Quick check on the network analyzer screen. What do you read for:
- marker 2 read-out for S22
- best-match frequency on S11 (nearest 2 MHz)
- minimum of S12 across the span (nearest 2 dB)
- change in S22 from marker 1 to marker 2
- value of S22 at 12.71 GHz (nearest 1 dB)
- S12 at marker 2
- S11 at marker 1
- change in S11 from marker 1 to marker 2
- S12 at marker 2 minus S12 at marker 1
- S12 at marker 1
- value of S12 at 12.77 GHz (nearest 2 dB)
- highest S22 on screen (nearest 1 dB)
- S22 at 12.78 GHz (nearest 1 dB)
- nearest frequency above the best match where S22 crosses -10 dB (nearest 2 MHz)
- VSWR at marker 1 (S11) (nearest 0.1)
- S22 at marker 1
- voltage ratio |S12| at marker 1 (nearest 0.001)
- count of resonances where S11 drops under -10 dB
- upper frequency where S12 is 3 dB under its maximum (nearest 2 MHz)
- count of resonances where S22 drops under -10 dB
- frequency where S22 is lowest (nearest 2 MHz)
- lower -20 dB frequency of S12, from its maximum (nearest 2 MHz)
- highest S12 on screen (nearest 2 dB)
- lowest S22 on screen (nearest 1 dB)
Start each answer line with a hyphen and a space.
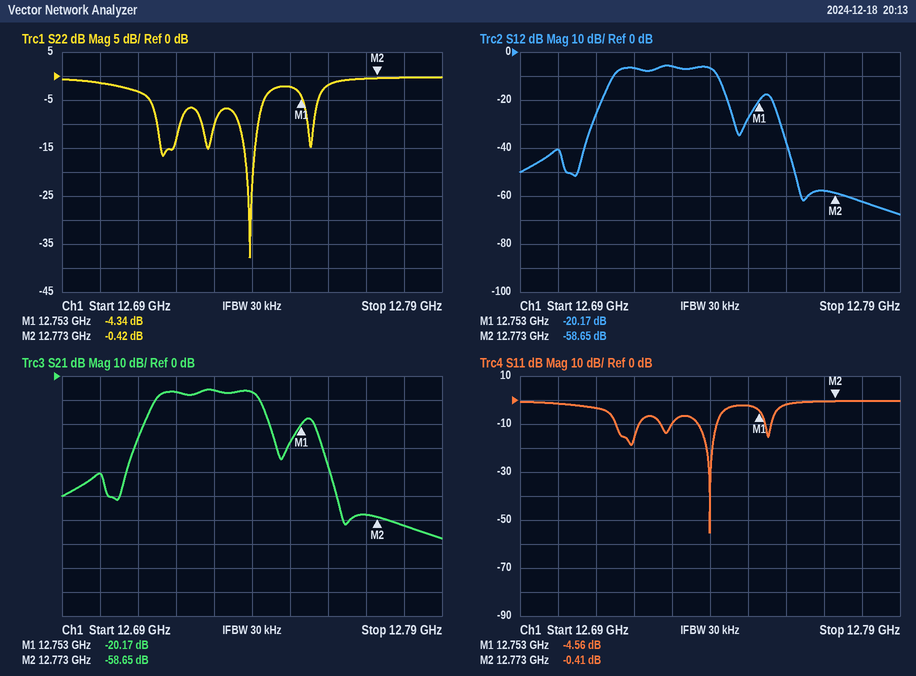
- -0.42 dB
- 12.740 GHz
- -68 dB
- 3.92 dB
- -3 dB
- -58.65 dB
- -4.56 dB
- 4.15 dB
- -38.48 dB
- -20.17 dB
- -58 dB
- 0 dB
- 0 dB
- 12.742 GHz
- 3.9
- -4.34 dB
- 0.098
- 4
- 12.742 GHz
- 4
- 12.740 GHz
- 12.710 GHz
- -6 dB
- -38 dB
